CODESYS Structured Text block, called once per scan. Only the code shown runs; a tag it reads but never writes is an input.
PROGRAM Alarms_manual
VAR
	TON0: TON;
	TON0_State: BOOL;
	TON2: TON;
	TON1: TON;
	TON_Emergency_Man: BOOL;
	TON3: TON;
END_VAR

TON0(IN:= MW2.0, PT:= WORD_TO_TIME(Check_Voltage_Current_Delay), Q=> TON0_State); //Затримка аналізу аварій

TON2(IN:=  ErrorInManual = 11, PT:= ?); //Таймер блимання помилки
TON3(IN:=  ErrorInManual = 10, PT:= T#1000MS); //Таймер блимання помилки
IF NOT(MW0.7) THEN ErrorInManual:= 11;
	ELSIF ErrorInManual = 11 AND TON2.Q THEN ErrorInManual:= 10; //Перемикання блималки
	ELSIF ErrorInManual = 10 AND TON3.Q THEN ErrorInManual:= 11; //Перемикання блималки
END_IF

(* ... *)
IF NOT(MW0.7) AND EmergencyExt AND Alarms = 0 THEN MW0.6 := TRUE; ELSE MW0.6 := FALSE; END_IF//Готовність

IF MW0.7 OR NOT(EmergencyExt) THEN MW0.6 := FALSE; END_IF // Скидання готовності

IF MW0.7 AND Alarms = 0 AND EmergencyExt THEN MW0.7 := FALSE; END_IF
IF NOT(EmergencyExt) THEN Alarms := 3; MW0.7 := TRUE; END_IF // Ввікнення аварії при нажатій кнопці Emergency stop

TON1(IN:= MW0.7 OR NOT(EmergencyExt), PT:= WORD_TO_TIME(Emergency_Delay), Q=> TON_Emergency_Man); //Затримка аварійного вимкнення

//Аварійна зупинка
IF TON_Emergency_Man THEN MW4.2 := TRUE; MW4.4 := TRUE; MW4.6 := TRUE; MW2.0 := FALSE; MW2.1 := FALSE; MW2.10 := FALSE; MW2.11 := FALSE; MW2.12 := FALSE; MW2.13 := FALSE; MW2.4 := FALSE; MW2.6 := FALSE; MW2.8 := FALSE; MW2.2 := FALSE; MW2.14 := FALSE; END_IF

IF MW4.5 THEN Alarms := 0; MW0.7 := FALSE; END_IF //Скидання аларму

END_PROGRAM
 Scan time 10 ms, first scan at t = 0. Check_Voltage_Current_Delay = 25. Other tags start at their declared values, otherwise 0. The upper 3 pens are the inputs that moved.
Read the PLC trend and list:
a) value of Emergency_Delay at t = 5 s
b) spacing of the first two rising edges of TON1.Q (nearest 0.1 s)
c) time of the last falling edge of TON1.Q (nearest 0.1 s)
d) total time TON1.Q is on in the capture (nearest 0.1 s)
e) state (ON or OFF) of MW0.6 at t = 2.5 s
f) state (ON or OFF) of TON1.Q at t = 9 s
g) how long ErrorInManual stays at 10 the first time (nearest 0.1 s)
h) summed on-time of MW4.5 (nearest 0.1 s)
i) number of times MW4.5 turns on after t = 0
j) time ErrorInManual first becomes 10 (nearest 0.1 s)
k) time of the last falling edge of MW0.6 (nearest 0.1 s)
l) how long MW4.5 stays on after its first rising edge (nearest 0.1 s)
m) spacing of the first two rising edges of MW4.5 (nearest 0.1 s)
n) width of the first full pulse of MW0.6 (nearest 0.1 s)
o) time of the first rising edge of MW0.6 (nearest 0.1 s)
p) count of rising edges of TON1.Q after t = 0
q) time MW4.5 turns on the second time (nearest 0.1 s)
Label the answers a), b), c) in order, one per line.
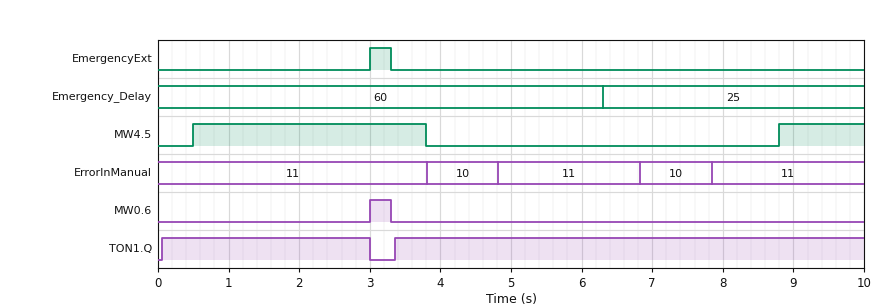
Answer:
a) 60
b) 3.3 s
c) 3.0 s
d) 9.6 s
e) OFF
f) ON
g) 1.0 s
h) 4.5 s
i) 2
j) 3.8 s
k) 3.3 s
l) 3.3 s
m) 8.3 s
n) 0.3 s
o) 3.0 s
p) 2
q) 8.8 s
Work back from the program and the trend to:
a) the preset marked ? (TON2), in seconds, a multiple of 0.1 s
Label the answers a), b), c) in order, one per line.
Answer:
a) 2.0 s
